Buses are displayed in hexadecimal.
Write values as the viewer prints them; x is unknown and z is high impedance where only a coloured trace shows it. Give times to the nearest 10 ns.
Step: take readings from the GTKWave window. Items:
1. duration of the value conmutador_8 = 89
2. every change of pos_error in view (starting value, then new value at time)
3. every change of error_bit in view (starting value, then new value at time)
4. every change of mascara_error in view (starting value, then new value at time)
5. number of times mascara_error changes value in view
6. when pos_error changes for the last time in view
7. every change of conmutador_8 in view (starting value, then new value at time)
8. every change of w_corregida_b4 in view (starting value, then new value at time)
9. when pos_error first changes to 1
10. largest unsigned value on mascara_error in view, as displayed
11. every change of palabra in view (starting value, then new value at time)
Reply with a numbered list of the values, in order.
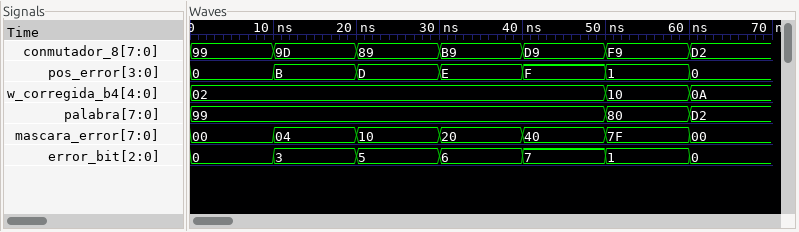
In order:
1. 10 ns
2. 0, B at 10 ns, D at 20 ns, E at 30 ns, F at 40 ns, 1 at 50 ns, 0 at 60 ns
3. 0, 3 at 10 ns, 5 at 20 ns, 6 at 30 ns, 7 at 40 ns, 1 at 50 ns, 0 at 60 ns
4. 00, 04 at 10 ns, 10 at 20 ns, 20 at 30 ns, 40 at 40 ns, 7F at 50 ns, 00 at 60 ns
5. 6
6. 60 ns
7. 99, 9D at 10 ns, 89 at 20 ns, B9 at 30 ns, D9 at 40 ns, F9 at 50 ns, D2 at 60 ns
8. 02, 10 at 50 ns, 0A at 60 ns
9. 50 ns
10. 7F
11. 99, 80 at 50 ns, D2 at 60 ns
